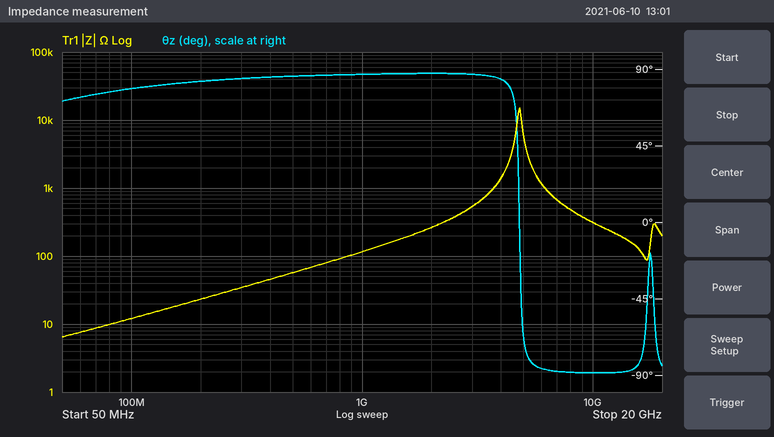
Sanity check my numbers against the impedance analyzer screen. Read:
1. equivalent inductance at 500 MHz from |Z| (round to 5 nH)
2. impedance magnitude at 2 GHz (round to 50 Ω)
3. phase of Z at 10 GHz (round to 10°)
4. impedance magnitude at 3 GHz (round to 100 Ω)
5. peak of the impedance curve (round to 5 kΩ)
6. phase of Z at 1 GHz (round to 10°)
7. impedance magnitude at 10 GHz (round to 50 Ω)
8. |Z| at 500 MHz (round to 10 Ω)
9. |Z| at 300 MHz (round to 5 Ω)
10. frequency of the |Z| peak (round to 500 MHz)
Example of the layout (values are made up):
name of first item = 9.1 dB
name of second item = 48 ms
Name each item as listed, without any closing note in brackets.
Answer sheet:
equivalent inductance at 500 MHz from |Z| = 20 nH
impedance magnitude at 2 GHz = 250 Ω
phase of Z at 10 GHz = -90°
impedance magnitude at 3 GHz = 500 Ω
peak of the impedance curve = 15 kΩ
phase of Z at 1 GHz = 90°
impedance magnitude at 10 GHz = 300 Ω
|Z| at 500 MHz = 60 Ω
|Z| at 300 MHz = 35 Ω
frequency of the |Z| peak = 5.0 GHz
